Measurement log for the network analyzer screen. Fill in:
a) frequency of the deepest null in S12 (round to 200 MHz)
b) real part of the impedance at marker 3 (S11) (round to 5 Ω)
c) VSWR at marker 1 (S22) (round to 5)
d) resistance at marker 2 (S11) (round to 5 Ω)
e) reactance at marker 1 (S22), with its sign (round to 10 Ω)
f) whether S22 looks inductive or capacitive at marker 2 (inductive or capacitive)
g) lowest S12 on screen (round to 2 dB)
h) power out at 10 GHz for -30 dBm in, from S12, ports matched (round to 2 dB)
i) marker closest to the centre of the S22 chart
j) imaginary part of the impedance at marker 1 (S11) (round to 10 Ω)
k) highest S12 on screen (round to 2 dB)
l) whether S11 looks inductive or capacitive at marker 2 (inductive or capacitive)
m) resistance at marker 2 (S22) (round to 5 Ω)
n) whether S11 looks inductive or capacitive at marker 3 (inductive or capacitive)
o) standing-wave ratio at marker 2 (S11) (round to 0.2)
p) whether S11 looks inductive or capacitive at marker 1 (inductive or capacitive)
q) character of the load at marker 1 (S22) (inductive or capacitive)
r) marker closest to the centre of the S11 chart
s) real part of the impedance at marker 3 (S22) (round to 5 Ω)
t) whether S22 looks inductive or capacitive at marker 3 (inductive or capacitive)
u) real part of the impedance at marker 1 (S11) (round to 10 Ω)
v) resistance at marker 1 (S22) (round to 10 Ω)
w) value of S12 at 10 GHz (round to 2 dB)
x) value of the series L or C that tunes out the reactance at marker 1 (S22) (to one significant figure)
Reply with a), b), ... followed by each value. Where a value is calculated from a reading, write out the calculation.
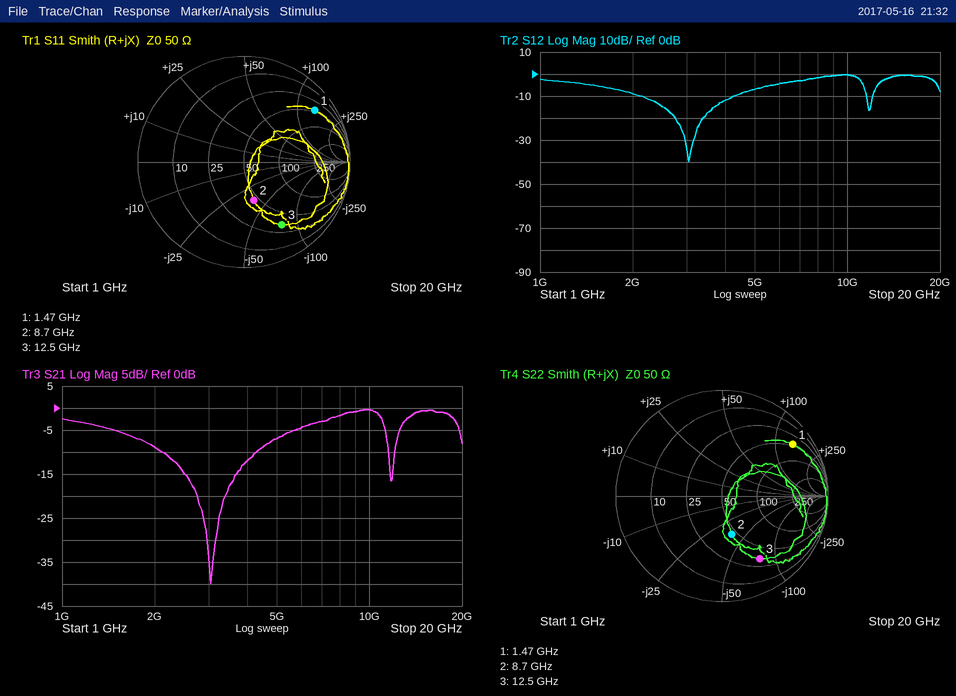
a) 3.0 GHz
b) 35 Ω
c) 10
d) 45 Ω
e) +140 Ω
f) capacitive
g) -40 dB
h) -30 dBm + (0 dB) = -30 dBm
i) marker 2
j) +140 Ω
k) 0 dB
l) capacitive
m) 45 Ω
n) capacitive
o) 2.2
p) inductive
q) inductive
r) marker 2
s) 35 Ω
t) capacitive
u) 50 Ω
v) 50 Ω
w) 0 dB
x) C = 1/(2π × 1.47 GHz × 140 Ω) ≈ 773 fF, so 800 fF to one significant figure
